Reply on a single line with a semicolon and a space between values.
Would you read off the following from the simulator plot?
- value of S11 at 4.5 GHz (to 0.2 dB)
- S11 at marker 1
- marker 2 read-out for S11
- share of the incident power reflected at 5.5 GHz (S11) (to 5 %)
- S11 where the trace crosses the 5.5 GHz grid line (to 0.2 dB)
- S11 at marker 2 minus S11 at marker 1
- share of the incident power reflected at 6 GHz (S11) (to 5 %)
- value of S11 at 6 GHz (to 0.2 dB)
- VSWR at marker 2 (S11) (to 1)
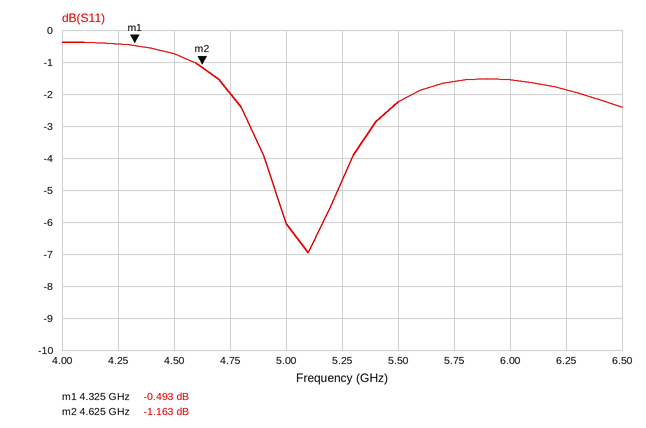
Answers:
-0.8 dB; -0.493 dB; -1.163 dB; 60 %; -2.2 dB; -0.670 dB; 70 %; -1.6 dB; 15
